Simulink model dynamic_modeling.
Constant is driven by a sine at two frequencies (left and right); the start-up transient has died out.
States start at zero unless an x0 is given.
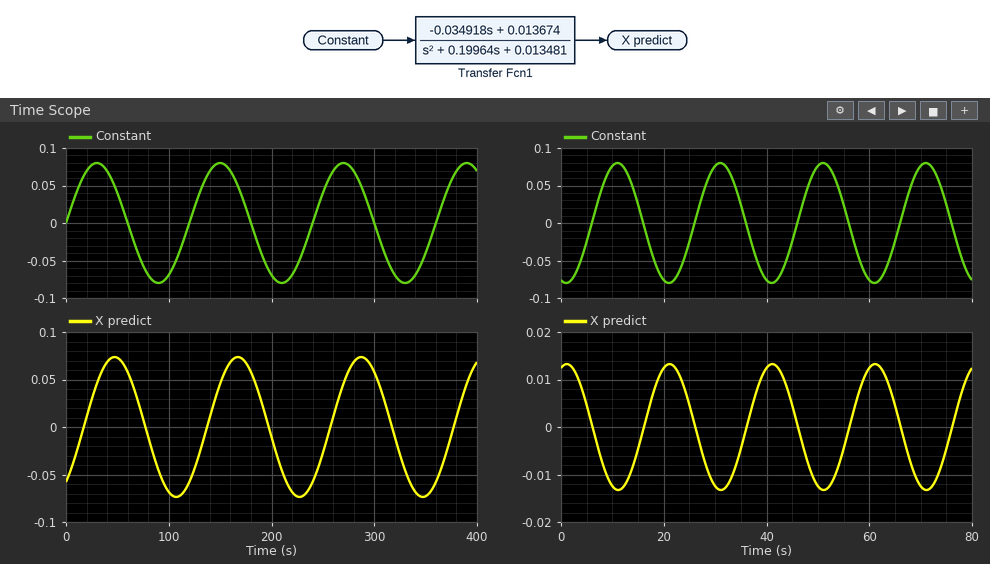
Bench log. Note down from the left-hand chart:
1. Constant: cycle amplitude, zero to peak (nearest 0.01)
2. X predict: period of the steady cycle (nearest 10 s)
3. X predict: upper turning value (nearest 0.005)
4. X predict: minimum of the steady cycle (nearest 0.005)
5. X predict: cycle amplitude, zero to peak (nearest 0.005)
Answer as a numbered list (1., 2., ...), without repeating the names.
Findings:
1. 0.08
2. 120 s
3. 0.075
4. -0.075
5. 0.075
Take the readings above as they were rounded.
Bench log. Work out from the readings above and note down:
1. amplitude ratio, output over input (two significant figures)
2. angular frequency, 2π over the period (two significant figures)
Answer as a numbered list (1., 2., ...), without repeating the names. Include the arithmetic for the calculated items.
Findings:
1. 0.075 / 0.08 = 0.94
2. 2π / 120 = 0.052 rad/s
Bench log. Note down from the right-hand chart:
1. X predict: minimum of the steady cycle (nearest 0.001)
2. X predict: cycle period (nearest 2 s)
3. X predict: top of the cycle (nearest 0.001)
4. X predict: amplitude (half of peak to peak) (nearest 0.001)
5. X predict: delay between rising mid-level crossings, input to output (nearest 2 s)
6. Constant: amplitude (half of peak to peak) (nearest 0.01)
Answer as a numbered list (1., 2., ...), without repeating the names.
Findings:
1. -0.013
2. 20 s
3. 0.013
4. 0.013
5. 10 s
6. 0.08
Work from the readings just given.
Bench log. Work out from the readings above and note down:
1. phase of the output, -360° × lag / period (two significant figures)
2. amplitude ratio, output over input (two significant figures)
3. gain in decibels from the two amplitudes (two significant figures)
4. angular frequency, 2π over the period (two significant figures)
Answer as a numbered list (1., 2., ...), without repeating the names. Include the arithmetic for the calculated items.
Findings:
1. -360 × 10 / 20 = -180°
2. 0.013 / 0.08 = 0.16
3. 20 log10(0.013 / 0.08) = -16 dB
4. 2π / 20 = 0.31 rad/s
